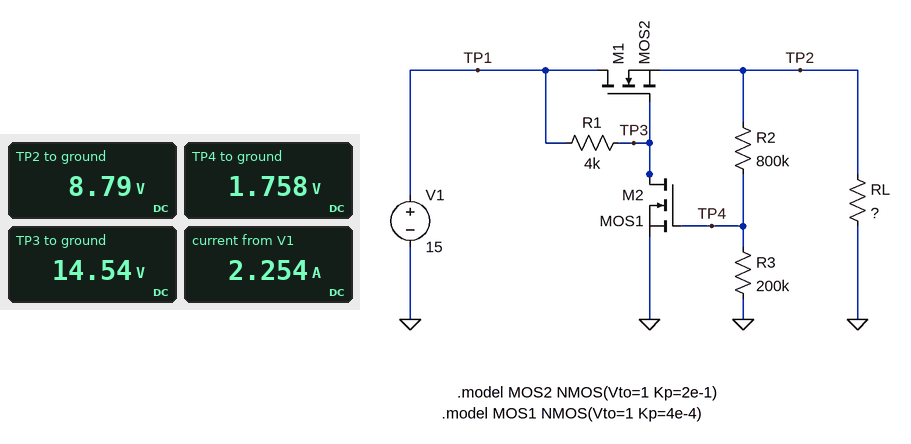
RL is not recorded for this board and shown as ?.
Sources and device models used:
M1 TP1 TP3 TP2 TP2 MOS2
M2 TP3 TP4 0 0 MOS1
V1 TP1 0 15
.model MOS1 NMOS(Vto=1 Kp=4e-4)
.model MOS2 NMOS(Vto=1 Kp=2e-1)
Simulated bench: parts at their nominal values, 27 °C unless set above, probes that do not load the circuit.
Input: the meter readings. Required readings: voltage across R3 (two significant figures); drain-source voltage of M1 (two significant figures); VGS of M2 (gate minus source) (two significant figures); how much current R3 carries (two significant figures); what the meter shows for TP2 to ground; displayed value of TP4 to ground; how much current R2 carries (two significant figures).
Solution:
1.8 V
6.2 V
1.8 V
8.8 µA
8.79 V
1.758 V
8.8 µA
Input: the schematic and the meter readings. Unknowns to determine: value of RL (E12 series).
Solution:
3.9 Ω
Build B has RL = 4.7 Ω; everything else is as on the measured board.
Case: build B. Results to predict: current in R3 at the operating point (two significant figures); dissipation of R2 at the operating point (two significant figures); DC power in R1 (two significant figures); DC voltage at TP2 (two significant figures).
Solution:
9.1 µA
66 µW
71 µW
9.1 V
